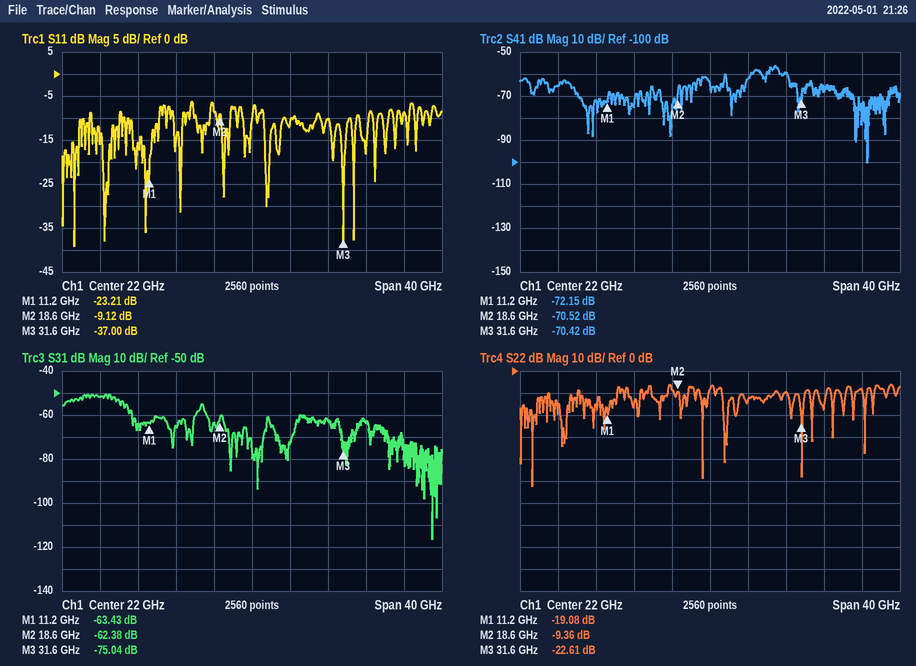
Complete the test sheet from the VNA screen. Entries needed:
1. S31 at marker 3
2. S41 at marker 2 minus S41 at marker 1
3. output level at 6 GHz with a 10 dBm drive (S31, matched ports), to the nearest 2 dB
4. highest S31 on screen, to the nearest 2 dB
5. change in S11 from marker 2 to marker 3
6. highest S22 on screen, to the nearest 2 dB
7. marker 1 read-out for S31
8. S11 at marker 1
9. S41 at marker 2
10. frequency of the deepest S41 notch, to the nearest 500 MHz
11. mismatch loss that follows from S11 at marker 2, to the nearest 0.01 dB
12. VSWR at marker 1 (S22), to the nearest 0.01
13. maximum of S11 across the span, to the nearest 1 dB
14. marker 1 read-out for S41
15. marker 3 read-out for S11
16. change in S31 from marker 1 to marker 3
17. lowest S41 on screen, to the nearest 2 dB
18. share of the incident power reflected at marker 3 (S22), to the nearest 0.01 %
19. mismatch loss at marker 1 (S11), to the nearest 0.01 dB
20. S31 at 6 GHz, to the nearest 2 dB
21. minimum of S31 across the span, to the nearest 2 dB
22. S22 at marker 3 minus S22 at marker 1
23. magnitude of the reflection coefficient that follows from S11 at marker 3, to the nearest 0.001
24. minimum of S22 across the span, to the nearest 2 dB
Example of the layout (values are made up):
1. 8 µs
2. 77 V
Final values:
1. -75.04 dB
2. 1.63 dB
3. -42 dBm
4. -50 dB
5. -27.88 dB
6. -6 dB
7. -63.43 dB
8. -23.21 dB
9. -70.52 dB
10. 38.5 GHz
11. 0.57 dB
12. 1.25
13. -6 dB
14. -72.15 dB
15. -37.00 dB
16. -11.61 dB
17. -100 dB
18. 0.55 %
19. 0.02 dB
20. -52 dB
21. -116 dB
22. -3.53 dB
23. 0.014
24. -52 dB
